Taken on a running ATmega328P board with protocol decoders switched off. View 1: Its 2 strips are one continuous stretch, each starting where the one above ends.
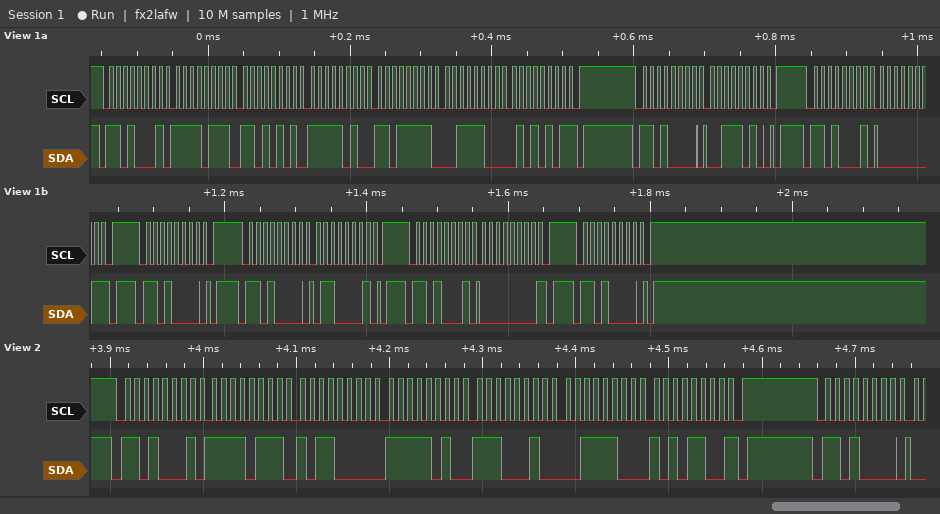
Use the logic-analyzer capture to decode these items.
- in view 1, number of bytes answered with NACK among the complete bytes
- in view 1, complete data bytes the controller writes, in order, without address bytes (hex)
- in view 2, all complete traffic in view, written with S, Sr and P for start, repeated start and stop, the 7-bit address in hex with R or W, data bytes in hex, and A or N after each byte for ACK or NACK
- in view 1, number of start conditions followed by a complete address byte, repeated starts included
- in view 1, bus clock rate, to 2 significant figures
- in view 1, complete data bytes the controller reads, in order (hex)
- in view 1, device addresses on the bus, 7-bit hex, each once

3
3A 61
S 68R A F7 A B0 A FA A E2 A 3C A AC N P S 68W A
7
100 kHz
F7 D5 FA DF 3C 55 01 00
0x68
